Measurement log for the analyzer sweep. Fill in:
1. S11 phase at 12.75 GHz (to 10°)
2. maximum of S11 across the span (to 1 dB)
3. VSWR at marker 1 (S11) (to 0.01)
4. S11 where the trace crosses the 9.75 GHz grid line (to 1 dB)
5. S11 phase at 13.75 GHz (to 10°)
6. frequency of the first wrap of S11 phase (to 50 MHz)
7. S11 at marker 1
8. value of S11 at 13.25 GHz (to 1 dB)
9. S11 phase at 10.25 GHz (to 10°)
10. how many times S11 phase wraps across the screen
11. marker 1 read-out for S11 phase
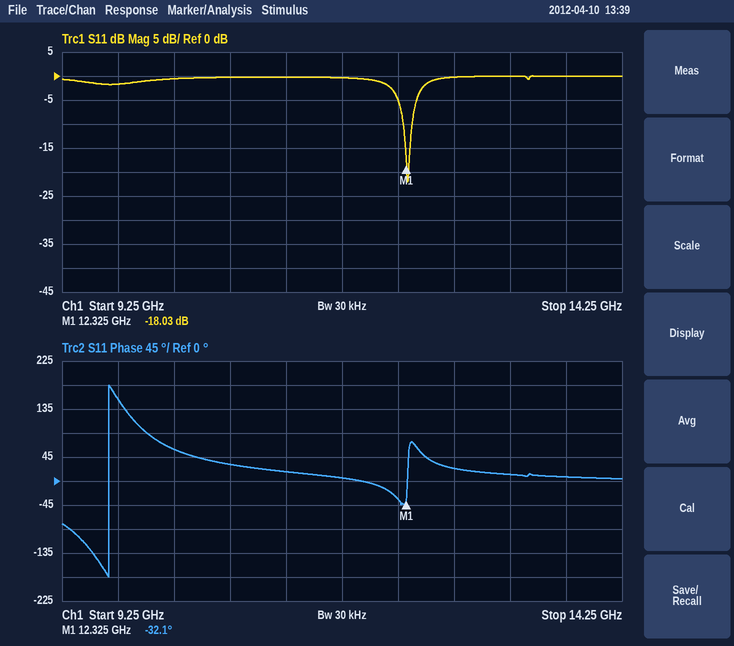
20°
0 dB
1.29
-2 dB
10°
9.65 GHz
-18.03 dB
0 dB
60°
1
-32.1°
